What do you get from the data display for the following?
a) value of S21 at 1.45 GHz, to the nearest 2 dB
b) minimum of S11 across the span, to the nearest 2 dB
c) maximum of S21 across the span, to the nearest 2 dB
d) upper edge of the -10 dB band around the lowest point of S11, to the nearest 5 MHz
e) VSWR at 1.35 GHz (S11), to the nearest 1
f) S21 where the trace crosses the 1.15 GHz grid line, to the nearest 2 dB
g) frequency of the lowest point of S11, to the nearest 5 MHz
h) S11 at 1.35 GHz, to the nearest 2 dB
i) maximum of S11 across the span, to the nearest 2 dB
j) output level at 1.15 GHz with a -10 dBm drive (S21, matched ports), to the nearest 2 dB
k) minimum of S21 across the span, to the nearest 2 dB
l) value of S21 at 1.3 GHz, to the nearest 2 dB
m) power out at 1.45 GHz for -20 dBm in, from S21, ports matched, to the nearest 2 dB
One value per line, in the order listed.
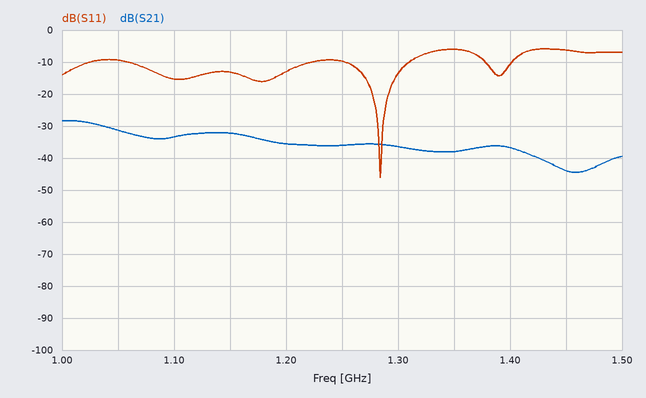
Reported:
-44 dB
-46 dB
-28 dB
1.310 GHz
3
-32 dB
1.285 GHz
-6 dB
-6 dB
-42 dBm
-44 dB
-36 dB
-64 dBm
